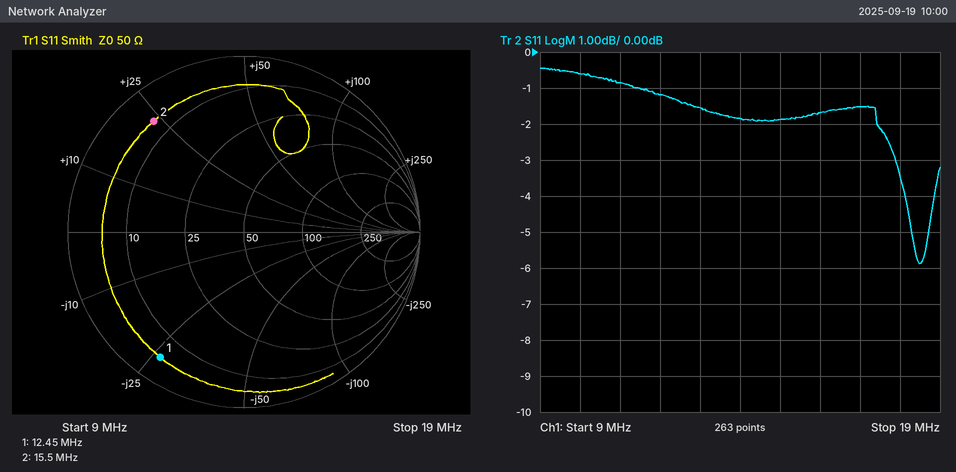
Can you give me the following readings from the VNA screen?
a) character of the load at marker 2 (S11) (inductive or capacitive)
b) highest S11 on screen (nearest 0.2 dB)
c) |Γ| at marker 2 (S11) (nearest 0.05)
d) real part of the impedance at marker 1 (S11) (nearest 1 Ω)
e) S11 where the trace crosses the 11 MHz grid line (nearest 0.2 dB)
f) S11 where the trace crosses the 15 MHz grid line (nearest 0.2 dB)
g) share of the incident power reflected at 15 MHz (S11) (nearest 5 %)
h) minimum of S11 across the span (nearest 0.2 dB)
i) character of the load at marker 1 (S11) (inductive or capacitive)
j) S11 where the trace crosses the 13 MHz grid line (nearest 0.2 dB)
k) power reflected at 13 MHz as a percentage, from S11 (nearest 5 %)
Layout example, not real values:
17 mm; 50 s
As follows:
inductive; -0.4 dB; 0.80; 5 Ω; -0.8 dB; -1.8 dB; 65 %; -5.8 dB; capacitive; -1.6 dB; 70 %
